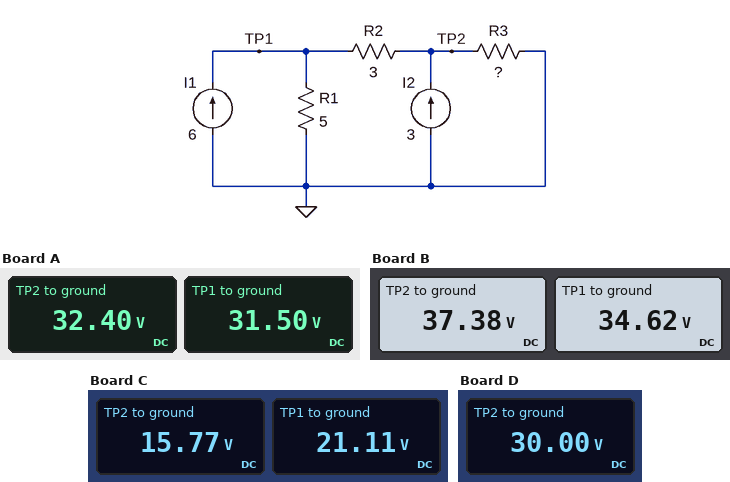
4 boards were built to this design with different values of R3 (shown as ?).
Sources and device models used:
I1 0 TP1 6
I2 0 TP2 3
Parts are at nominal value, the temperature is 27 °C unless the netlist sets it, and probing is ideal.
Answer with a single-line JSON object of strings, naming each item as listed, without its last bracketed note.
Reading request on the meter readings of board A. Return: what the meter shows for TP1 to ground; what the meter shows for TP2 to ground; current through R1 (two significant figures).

{"what the meter shows for TP1 to ground": "31.50 V", "what the meter shows for TP2 to ground": "32.40 V", "current through R1": "6.3 A"}
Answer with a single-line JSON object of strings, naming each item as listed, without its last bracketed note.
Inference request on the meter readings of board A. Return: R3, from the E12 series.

{"R3, from the E12 series": "12 Ω"}
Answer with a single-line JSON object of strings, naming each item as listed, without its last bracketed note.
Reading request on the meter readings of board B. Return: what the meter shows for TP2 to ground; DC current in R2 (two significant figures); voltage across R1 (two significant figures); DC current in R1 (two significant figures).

{"what the meter shows for TP2 to ground": "37.38 V", "DC current in R2": "920 mA", "voltage across R1": "35 V", "DC current in R1": "6.9 A"}
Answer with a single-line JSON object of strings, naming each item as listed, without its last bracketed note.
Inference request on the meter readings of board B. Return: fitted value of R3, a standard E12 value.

{"fitted value of R3, a standard E12 value": "18 Ω"}
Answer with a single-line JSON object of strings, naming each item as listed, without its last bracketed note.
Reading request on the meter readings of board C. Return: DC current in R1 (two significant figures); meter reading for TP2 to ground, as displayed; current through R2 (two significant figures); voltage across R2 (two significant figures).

{"DC current in R1": "4.2 A", "meter reading for TP2 to ground, as displayed": "15.77 V", "current through R2": "1.8 A", "voltage across R2": "5.3 V"}
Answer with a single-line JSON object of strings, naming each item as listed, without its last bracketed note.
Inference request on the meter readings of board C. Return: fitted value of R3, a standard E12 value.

{"fitted value of R3, a standard E12 value": "3.3 Ω"}
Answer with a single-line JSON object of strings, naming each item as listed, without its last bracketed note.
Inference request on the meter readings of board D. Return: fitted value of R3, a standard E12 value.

{"fitted value of R3, a standard E12 value": "10 Ω"}
